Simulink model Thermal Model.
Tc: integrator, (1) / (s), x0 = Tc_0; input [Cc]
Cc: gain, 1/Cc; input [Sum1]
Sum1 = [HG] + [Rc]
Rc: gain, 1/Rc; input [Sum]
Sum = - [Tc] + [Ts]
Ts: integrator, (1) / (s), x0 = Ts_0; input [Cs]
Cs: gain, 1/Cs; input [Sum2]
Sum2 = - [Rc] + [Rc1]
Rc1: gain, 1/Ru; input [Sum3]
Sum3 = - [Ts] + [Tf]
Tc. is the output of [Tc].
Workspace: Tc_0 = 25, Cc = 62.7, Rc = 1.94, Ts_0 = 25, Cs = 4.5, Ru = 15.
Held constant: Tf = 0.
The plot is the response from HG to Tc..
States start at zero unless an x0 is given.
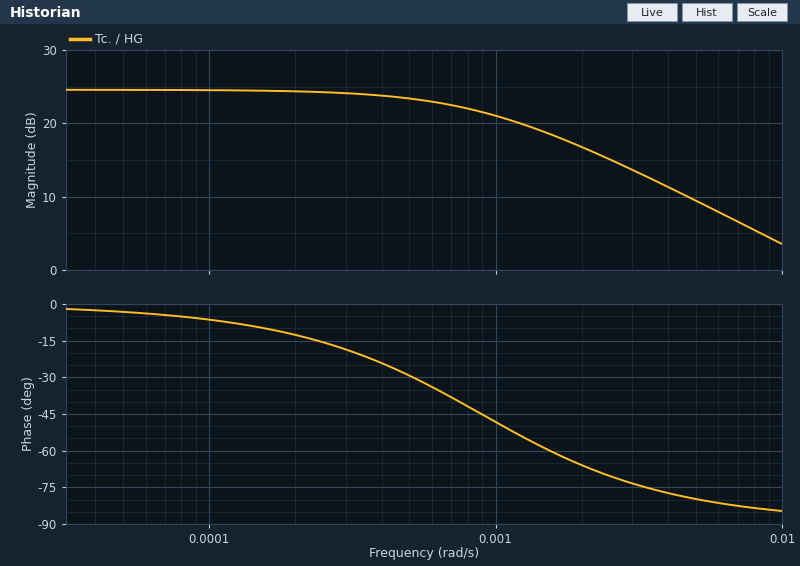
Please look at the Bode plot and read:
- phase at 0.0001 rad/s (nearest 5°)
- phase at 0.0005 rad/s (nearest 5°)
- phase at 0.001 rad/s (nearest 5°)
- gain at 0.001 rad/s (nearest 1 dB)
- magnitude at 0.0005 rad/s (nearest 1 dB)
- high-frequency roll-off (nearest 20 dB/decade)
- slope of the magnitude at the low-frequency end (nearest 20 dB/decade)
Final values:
-5°
-30°
-50°
21 dB
23 dB
-20 dB/decade
0 dB/decade
